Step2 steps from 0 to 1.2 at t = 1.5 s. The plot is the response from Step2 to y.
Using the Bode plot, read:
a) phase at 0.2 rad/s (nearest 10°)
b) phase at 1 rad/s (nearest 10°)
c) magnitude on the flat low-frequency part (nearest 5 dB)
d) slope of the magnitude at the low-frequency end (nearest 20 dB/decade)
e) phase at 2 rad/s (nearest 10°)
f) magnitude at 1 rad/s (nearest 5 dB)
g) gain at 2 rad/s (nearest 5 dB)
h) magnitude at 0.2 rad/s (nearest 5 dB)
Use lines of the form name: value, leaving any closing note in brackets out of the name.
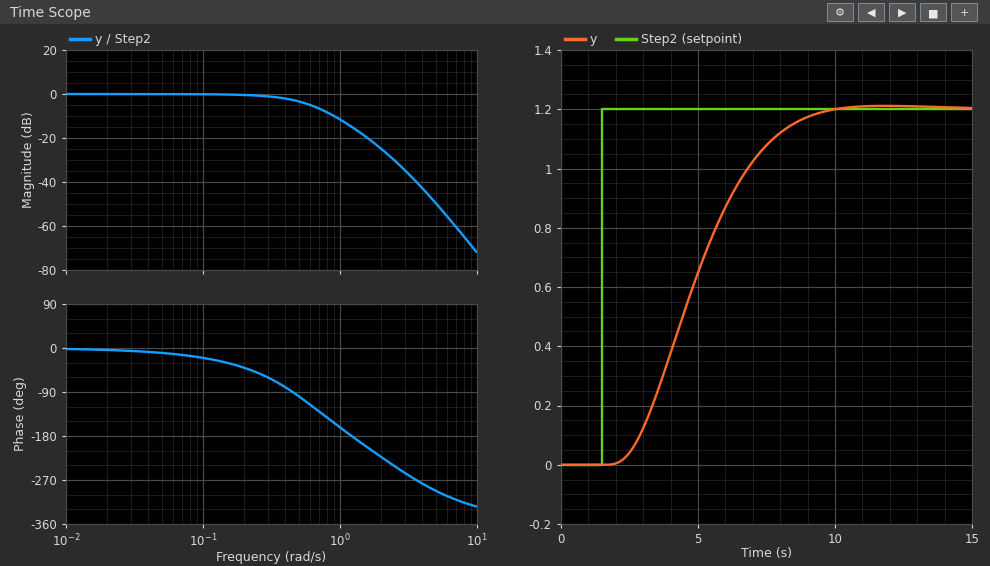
phase at 0.2 rad/s: -40°
phase at 1 rad/s: -160°
magnitude on the flat low-frequency part: 0 dB
slope of the magnitude at the low-frequency end: 0 dB/decade
phase at 2 rad/s: -220°
magnitude at 1 rad/s: -10 dB
gain at 2 rad/s: -25 dB
magnitude at 0.2 rad/s: 0 dB
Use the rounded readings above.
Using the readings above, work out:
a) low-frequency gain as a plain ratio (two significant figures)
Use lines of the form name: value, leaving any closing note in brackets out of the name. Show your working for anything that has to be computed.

low-frequency gain as a plain ratio: 10^(0 / 20) = 1.0
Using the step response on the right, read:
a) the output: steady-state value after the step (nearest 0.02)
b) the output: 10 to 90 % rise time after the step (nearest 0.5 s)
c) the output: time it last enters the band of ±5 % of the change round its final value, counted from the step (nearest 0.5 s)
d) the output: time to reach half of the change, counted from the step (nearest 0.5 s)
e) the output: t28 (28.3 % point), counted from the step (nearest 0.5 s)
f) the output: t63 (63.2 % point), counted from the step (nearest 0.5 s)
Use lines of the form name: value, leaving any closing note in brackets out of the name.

the output: steady-state value after the step: 1.20
the output: 10 to 90 % rise time after the step: 4.5 s
the output: time it last enters the band of ±5 % of the change round its final value, counted from the step: 7.0 s
the output: time to reach half of the change, counted from the step: 3.5 s
the output: t28 (28.3 % point), counted from the step: 2.5 s
the output: t63 (63.2 % point), counted from the step: 4.0 s
